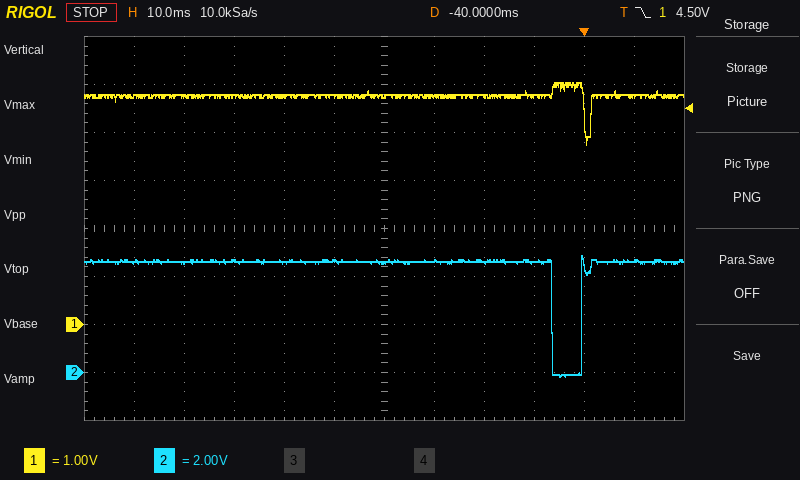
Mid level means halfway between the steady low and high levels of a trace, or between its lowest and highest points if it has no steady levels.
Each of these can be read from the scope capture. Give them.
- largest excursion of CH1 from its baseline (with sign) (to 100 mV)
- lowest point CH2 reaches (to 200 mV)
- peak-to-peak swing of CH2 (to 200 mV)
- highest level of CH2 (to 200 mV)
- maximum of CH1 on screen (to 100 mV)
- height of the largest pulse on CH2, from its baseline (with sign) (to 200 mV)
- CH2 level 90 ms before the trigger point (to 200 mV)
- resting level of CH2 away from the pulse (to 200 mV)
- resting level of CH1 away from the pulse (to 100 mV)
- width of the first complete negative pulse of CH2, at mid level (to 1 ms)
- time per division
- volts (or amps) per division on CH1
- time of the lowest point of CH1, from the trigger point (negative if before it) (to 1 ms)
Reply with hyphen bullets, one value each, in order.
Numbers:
- -1.0 V
- -200 mV
- 5.0 V
- 4.8 V
- 5.0 V
- -4.8 V
- 4.6 V
- 4.6 V
- 4.8 V
- 6 ms
- 10 ms
- 1 V
- +1 ms
